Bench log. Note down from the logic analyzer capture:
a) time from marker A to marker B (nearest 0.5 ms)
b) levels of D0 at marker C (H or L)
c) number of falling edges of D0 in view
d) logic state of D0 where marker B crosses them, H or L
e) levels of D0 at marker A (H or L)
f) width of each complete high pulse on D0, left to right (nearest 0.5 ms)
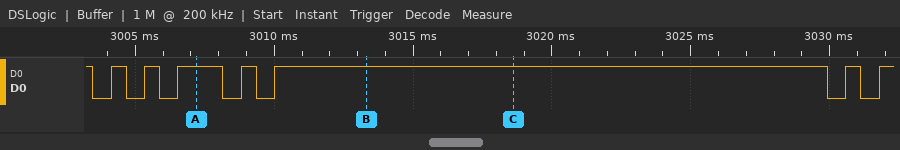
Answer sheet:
6 ms
D0=H
7
D0=H
D0=H
0.5 ms, 0.5 ms, 1.5 ms, 0.5 ms, 20 ms, 0.5 ms
